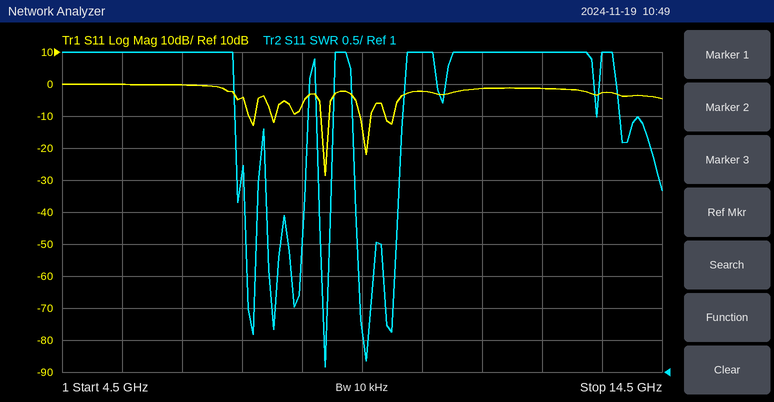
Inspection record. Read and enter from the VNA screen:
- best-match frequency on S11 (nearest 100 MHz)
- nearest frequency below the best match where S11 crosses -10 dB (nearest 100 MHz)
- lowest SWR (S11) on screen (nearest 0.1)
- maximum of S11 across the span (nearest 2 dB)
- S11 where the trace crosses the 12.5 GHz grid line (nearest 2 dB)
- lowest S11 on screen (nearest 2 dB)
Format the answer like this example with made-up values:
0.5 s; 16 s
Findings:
8.9 GHz; 8.8 GHz; 1.1; 0 dB; -2 dB; -28 dB
